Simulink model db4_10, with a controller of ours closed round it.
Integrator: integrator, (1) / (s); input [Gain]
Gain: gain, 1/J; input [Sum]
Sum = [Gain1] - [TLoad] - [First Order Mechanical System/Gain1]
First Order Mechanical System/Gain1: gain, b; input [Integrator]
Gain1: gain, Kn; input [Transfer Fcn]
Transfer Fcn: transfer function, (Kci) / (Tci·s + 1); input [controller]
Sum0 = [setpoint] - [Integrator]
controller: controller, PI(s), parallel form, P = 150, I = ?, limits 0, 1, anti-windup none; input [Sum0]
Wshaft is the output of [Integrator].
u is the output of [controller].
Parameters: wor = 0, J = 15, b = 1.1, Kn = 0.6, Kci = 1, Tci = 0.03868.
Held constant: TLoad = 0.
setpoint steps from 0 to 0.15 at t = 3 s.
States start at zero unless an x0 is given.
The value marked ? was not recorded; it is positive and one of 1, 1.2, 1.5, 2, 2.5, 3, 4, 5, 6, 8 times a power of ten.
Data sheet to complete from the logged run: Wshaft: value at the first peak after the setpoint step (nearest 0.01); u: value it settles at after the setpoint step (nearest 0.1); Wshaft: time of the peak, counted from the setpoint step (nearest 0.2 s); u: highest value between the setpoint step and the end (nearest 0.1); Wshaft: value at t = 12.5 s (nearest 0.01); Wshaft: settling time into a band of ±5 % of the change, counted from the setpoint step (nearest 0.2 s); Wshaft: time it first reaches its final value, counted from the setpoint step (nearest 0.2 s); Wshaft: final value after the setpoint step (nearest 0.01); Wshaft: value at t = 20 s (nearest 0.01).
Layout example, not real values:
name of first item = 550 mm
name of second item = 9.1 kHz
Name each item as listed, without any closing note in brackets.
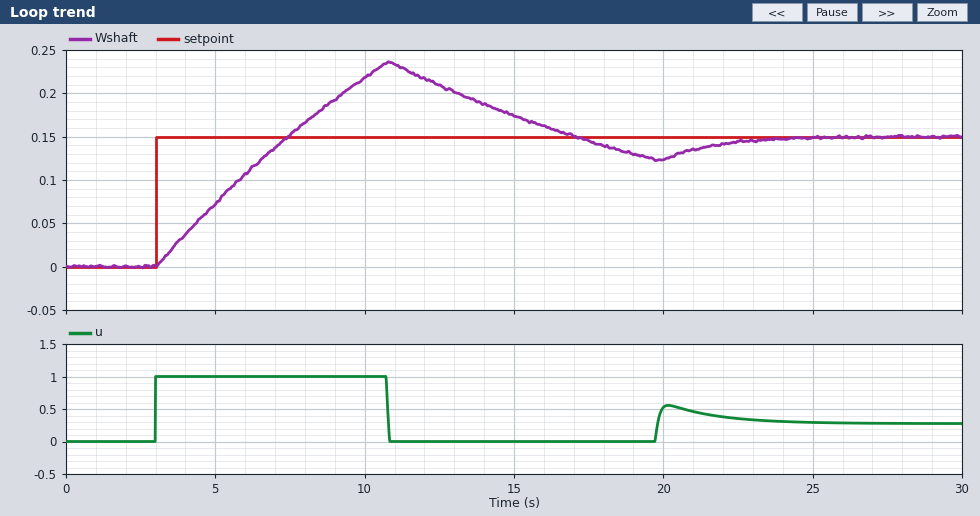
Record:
Wshaft: value at the first peak after the setpoint step = 0.24
u: value it settles at after the setpoint step = 0.3
Wshaft: time of the peak, counted from the setpoint step = 7.8 s
u: highest value between the setpoint step and the end = 1.0
Wshaft: value at t = 12.5 s = 0.21
Wshaft: settling time into a band of ±5 % of the change, counted from the setpoint step = 19.2 s
Wshaft: time it first reaches its final value, counted from the setpoint step = 4.4 s
Wshaft: final value after the setpoint step = 0.15
Wshaft: value at t = 20 s = 0.12
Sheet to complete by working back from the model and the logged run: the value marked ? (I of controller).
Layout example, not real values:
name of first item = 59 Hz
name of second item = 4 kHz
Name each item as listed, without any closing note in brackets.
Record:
the value marked ? = 80
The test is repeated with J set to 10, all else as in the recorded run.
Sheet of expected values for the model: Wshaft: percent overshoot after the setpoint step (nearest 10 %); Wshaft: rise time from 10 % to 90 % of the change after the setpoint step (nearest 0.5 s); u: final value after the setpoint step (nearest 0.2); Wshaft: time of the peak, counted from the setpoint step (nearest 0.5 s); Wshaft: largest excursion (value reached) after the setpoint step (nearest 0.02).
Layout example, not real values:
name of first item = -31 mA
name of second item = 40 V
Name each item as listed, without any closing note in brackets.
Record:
Wshaft: percent overshoot after the setpoint step = 50 %
Wshaft: rise time from 10 % to 90 % of the change after the setpoint step = 2.5 s
u: final value after the setpoint step = 0.2
Wshaft: time of the peak, counted from the setpoint step = 5.0 s
Wshaft: largest excursion (value reached) after the setpoint step = 0.22
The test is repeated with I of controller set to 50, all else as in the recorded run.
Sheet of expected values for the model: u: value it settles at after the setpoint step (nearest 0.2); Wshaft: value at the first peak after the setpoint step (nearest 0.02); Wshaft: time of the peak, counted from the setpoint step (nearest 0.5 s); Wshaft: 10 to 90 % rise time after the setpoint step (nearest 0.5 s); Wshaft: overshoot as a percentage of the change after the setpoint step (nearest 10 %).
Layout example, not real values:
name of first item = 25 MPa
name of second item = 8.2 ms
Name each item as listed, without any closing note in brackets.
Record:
u: value it settles at after the setpoint step = 0.2
Wshaft: value at the first peak after the setpoint step = 0.22
Wshaft: time of the peak, counted from the setpoint step = 7.0 s
Wshaft: 10 to 90 % rise time after the setpoint step = 3.5 s
Wshaft: overshoot as a percentage of the change after the setpoint step = 50 %
